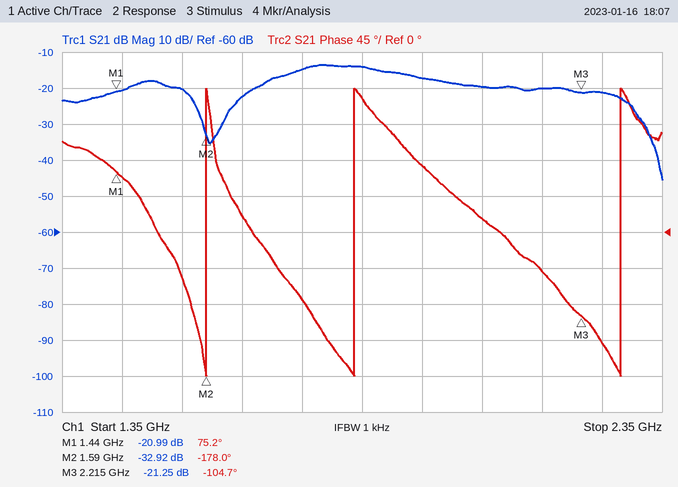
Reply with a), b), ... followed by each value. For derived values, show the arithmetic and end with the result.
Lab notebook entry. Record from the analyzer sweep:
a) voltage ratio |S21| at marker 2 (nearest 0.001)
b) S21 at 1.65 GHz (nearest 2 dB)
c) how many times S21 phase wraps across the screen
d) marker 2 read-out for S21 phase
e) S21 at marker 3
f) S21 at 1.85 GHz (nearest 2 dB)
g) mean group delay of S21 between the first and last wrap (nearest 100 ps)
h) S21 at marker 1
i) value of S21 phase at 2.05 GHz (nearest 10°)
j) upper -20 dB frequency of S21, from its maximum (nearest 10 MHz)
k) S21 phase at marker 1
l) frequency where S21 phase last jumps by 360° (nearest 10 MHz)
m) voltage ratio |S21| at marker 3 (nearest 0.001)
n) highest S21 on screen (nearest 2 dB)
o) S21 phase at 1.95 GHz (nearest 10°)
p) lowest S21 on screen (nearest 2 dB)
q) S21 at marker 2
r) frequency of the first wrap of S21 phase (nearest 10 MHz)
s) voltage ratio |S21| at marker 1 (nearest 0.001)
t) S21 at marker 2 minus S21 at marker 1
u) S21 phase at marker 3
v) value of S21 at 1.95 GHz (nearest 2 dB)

a) 10^(-32.92/20) ≈ 0.023
b) -22 dB
c) 3
d) -178.0°
e) -21.25 dB
f) -14 dB
g) 2 cycles / (2.28 GHz − 1.59 GHz) ≈ 2.9 ns
h) -20.99 dB
i) 20°
j) 2.33 GHz
k) 75.2°
l) 2.28 GHz
m) 10^(-21.25/20) ≈ 0.087
n) -14 dB
o) 80°
p) -46 dB
q) -32.92 dB
r) 1.59 GHz
s) 10^(-20.99/20) ≈ 0.089
t) -32.92 − (-20.99) = -11.93 dB
u) -104.7°
v) -18 dB
